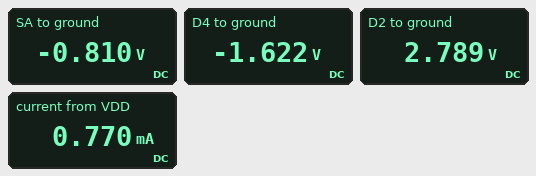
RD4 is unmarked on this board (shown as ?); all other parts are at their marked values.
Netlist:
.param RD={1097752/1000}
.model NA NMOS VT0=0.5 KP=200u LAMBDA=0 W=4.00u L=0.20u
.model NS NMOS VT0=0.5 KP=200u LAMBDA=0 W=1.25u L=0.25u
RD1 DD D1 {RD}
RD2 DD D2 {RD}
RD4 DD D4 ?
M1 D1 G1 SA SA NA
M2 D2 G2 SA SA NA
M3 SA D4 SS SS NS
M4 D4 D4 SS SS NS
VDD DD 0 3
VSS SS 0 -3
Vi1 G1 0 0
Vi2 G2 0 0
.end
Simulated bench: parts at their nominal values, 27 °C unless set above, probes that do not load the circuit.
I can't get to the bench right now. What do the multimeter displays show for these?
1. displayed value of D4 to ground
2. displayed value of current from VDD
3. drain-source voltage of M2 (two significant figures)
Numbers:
-1.622 V
0.770 mA
3.6 V
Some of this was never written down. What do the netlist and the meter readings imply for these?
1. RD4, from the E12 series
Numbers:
12 kΩ
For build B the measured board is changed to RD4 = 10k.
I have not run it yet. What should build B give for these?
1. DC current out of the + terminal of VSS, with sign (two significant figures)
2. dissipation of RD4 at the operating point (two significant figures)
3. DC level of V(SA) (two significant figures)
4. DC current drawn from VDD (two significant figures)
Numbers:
-910 µA
2.1 mW
-840 mV
910 µA
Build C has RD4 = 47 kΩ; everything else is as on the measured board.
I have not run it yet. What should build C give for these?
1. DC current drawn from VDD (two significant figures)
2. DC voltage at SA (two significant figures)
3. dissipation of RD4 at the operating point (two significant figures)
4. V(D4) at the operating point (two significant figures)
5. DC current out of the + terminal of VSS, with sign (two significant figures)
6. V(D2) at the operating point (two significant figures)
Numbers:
210 µA
-660 mV
540 µW
-2.0 V
-210 µA
2.9 V
